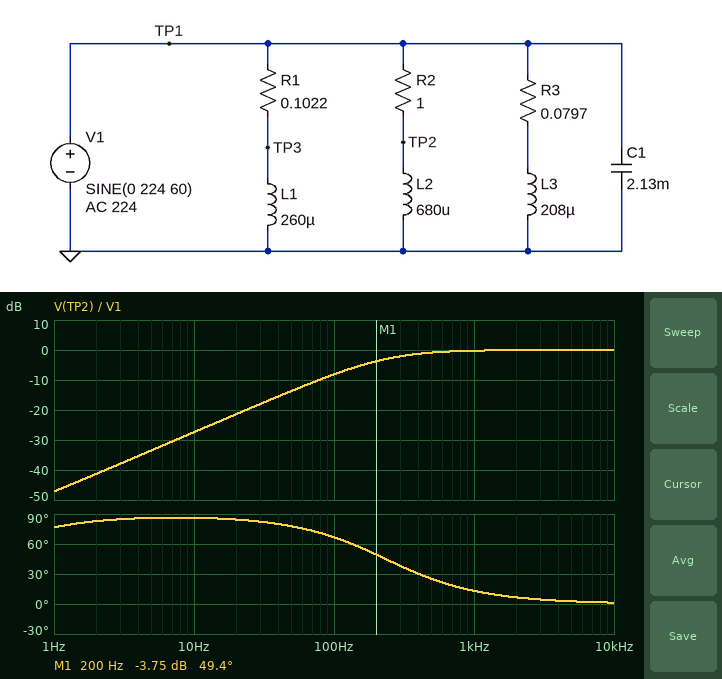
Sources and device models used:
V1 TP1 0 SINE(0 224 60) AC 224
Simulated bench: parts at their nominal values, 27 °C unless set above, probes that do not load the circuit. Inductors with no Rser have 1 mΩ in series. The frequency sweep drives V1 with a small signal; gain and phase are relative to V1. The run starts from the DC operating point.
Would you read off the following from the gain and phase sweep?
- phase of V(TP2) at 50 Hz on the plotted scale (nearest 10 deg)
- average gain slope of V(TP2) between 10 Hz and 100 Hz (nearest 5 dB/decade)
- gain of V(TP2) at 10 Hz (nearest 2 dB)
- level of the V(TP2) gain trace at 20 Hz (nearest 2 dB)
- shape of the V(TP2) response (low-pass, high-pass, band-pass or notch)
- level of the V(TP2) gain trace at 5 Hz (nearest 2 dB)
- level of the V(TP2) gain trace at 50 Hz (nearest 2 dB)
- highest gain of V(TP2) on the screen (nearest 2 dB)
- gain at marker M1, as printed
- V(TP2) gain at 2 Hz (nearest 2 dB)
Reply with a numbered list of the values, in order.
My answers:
1. 80 deg
2. 20 dB/decade
3. -28 dB
4. -22 dB
5. high-pass
6. -34 dB
7. -14 dB
8. 0 dB
9. -3.75 dB
10. -42 dB
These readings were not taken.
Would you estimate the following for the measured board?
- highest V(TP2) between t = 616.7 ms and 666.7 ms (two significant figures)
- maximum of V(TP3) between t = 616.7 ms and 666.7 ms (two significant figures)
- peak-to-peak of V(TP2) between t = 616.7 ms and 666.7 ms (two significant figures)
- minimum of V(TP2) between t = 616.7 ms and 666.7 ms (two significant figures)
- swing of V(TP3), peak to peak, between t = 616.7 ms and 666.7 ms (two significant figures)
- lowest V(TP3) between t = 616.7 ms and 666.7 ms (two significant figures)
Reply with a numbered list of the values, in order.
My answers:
1. 56 V
2. 150 V
3. 110 V
4. -56 V
5. 310 V
6. -150 V
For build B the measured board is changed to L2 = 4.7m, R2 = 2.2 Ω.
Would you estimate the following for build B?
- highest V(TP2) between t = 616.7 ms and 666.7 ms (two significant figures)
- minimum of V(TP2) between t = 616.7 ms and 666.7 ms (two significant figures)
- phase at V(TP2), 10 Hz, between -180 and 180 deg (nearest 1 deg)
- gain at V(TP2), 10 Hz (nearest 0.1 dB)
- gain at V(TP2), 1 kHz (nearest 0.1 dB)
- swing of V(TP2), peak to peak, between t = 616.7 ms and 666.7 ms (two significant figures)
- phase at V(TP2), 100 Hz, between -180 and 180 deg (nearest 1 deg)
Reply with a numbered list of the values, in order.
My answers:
1. 140 V
2. -140 V
3. 82 deg
4. -17.5 dB
5. 0 dB
6. 280 V
7. 37 deg
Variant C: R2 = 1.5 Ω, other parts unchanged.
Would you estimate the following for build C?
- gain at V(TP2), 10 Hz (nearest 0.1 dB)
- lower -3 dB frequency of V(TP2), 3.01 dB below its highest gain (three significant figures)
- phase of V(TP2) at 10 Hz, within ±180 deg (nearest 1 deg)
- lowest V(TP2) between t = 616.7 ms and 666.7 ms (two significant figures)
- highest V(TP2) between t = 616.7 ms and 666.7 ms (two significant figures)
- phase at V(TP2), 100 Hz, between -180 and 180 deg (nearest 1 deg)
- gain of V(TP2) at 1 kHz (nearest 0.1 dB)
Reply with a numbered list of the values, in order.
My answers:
1. -30.9 dB
2. 351 Hz
3. 87 deg
4. -38 V
5. 38 V
6. 74 deg
7. -0.5 dB
